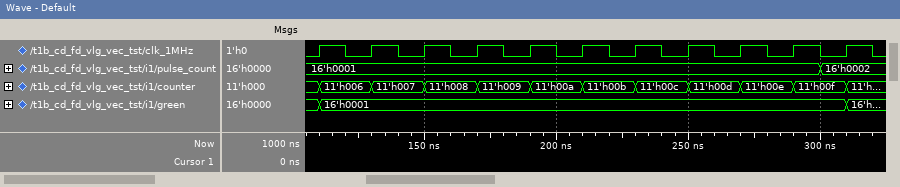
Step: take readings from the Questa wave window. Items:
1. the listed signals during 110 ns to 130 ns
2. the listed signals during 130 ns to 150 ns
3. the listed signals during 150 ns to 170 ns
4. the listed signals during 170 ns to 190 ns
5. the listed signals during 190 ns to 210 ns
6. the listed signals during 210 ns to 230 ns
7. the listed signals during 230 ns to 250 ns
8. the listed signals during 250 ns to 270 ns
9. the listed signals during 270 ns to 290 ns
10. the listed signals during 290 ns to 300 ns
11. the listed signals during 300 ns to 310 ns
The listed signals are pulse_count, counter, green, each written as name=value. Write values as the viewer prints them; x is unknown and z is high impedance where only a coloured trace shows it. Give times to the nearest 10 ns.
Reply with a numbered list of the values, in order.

1. pulse_count=16'h0001, counter=11'h006, green=16'h0001
2. pulse_count=16'h0001, counter=11'h007, green=16'h0001
3. pulse_count=16'h0001, counter=11'h008, green=16'h0001
4. pulse_count=16'h0001, counter=11'h009, green=16'h0001
5. pulse_count=16'h0001, counter=11'h00a, green=16'h0001
6. pulse_count=16'h0001, counter=11'h00b, green=16'h0001
7. pulse_count=16'h0001, counter=11'h00c, green=16'h0001
8. pulse_count=16'h0001, counter=11'h00d, green=16'h0001
9. pulse_count=16'h0001, counter=11'h00e, green=16'h0001
10. pulse_count=16'h0001, counter=11'h00f, green=16'h0001
11. pulse_count=16'h0002, counter=11'h00f, green=16'h0001
